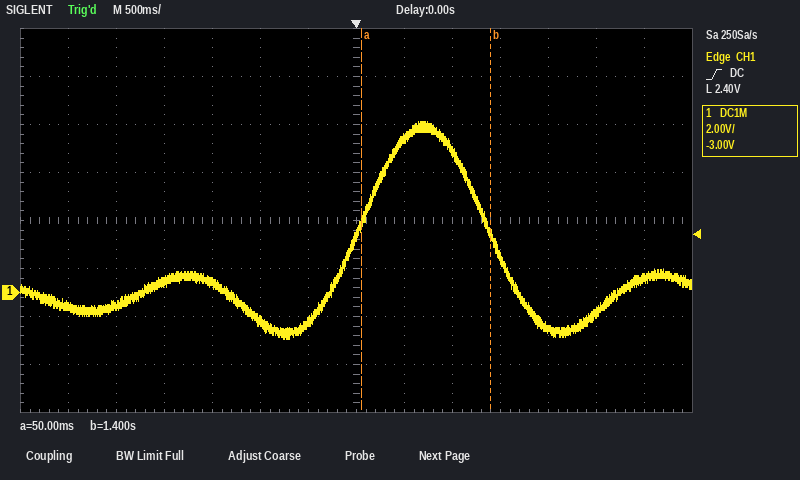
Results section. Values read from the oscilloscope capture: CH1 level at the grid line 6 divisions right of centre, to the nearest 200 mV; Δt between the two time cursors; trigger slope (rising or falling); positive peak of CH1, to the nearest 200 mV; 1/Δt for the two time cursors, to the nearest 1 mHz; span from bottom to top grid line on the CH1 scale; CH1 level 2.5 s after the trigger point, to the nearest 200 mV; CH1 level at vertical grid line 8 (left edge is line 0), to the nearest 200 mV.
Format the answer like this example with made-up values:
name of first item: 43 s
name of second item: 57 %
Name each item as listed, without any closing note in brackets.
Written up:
CH1 level at the grid line 6 divisions right of centre, to the nearest 200 mV: 600 mV
Δt between the two time cursors: 1.35 s
trigger slope: rising
positive peak of CH1, to the nearest 200 mV: 7.2 V
1/Δt for the two time cursors, to the nearest 1 mHz: 741 mHz
span from bottom to top grid line on the CH1 scale: 16 V
CH1 level 2.5 s after the trigger point, to the nearest 200 mV: -800 mV
CH1 level at vertical grid line 8 (left edge is line 0), to the nearest 200 mV: 6.4 V
